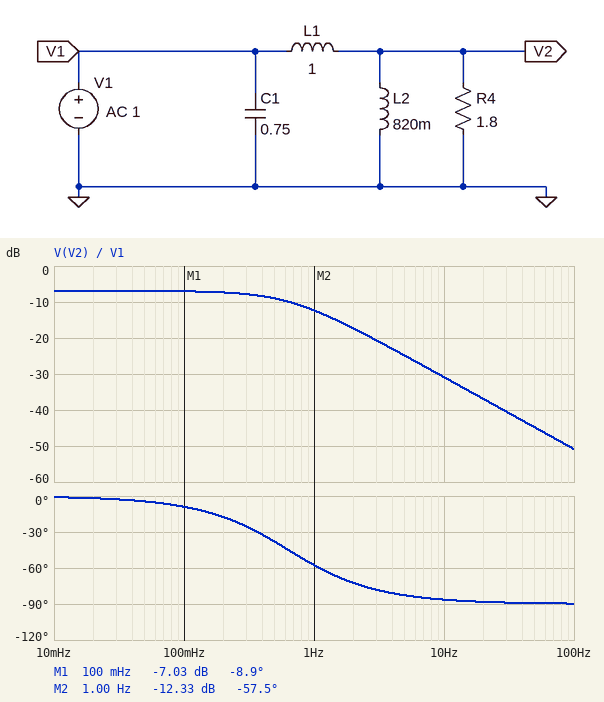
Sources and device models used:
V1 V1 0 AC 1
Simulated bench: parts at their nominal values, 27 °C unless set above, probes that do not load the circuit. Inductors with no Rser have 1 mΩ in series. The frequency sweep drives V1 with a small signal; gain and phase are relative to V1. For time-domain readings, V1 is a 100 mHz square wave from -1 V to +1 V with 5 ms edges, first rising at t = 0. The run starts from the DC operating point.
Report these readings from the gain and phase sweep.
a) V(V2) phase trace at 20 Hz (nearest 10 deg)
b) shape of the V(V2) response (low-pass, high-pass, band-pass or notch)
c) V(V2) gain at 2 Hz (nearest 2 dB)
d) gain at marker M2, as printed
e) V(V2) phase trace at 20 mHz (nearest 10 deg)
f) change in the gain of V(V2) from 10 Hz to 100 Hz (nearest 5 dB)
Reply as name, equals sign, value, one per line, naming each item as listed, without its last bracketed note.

V(V2) phase trace at 20 Hz = -90 deg
shape of the V(V2) response = low-pass
V(V2) gain at 2 Hz = -18 dB
gain at marker M2, as printed = -12.33 dB
V(V2) phase trace at 20 mHz = 0 deg
change in the gain of V(V2) from 10 Hz to 100 Hz = -20 dB
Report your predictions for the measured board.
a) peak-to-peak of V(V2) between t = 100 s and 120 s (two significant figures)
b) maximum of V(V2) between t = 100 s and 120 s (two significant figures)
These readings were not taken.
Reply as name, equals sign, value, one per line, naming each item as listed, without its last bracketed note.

peak-to-peak of V(V2) between t = 100 s and 120 s = 900 mV
maximum of V(V2) between t = 100 s and 120 s = 410 mV
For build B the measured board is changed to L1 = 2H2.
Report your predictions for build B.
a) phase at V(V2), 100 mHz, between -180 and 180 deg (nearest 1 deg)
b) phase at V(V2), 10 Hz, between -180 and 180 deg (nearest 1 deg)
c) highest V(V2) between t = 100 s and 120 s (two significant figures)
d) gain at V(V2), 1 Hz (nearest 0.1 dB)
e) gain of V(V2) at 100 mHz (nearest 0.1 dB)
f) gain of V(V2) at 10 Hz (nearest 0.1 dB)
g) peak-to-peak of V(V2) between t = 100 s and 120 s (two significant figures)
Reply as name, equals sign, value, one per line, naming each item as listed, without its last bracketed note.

phase at V(V2), 100 mHz, between -180 and 180 deg = -12 deg
phase at V(V2), 10 Hz, between -180 and 180 deg = -87 deg
highest V(V2) between t = 100 s and 120 s = 60 mV
gain at V(V2), 1 Hz = -18.6 dB
gain of V(V2) at 100 mHz = -11.5 dB
gain of V(V2) at 10 Hz = -37.7 dB
peak-to-peak of V(V2) between t = 100 s and 120 s = 550 mV
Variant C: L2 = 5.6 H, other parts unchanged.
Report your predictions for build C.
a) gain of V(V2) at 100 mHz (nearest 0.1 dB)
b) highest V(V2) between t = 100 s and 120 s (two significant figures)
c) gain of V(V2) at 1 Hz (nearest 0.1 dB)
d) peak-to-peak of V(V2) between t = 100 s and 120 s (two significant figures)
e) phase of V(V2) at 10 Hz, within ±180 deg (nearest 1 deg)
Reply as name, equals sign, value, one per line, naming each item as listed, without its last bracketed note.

gain of V(V2) at 100 mHz = -1.8 dB
highest V(V2) between t = 100 s and 120 s = 1.2 V
gain of V(V2) at 1 Hz = -11.3 dB
peak-to-peak of V(V2) between t = 100 s and 120 s = 1.7 V
phase of V(V2) at 10 Hz, within ±180 deg = -88 deg
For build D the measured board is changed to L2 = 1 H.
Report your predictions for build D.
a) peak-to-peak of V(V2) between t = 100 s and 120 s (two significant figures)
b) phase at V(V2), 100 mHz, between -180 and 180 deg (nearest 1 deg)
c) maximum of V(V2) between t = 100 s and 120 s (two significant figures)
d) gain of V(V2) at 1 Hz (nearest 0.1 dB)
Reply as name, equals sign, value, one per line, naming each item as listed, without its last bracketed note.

peak-to-peak of V(V2) between t = 100 s and 120 s = 1.0 V
phase at V(V2), 100 mHz, between -180 and 180 deg = -10 deg
maximum of V(V2) between t = 100 s and 120 s = 500 mV
gain of V(V2) at 1 Hz = -12.1 dB
